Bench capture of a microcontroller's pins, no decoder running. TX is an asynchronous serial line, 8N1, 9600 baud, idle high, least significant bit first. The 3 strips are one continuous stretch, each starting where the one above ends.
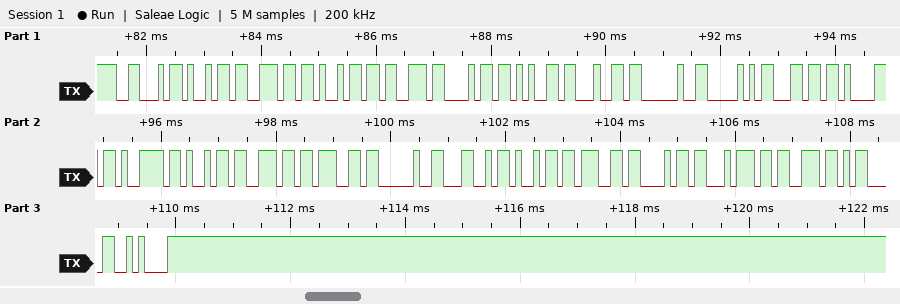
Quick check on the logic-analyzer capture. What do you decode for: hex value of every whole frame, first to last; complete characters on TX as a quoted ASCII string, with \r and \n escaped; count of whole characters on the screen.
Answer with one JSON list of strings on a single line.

["46 69 6E 69 73 68 65 64 20 50 6C 61 79 69 6E 67 20 4C 69 67 68 74 73 0D 0A", "\"Finished Playing Lights\\r\\n\"", "25"]
